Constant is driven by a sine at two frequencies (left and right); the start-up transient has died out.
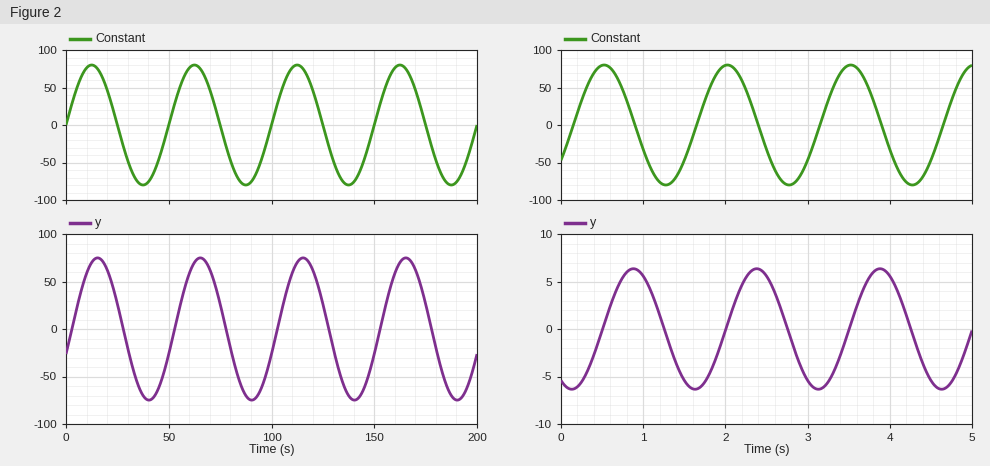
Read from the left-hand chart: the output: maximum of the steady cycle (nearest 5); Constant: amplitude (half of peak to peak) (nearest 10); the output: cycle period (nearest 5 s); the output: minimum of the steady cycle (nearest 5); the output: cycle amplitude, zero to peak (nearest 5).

75
80
50 s
-75
75
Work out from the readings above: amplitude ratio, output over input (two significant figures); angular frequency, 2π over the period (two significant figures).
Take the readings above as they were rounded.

0.94
0.13 rad/s
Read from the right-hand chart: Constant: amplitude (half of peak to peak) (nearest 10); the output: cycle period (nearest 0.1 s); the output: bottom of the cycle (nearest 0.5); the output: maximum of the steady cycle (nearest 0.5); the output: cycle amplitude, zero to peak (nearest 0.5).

80
1.5 s
-6.5
6.5
6.5
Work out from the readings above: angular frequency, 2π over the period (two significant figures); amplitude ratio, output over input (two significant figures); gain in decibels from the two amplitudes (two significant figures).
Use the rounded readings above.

4.2 rad/s
0.081
-22 dB
